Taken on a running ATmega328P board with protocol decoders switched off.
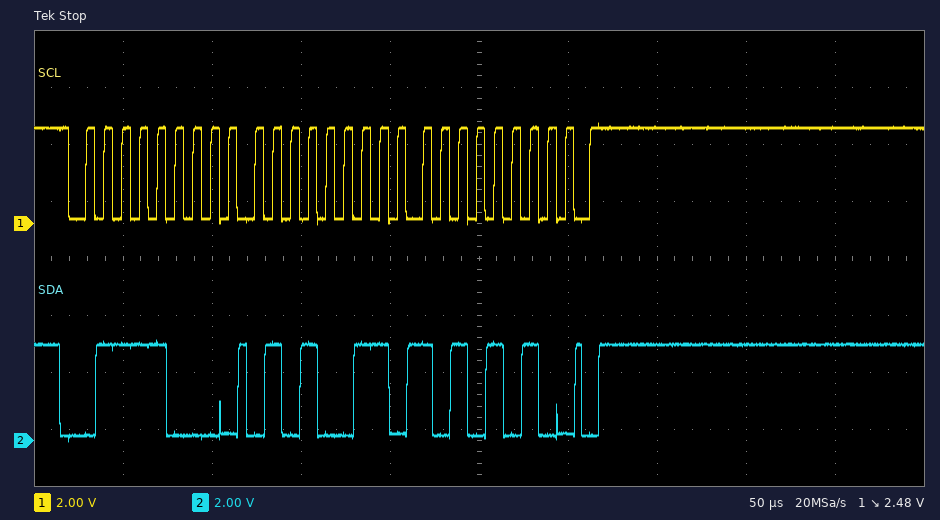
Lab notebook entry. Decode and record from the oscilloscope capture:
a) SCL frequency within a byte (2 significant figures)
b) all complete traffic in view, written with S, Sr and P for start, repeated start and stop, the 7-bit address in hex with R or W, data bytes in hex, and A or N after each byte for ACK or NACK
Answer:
100 kHz
S 3CW A 53 A AA A P
